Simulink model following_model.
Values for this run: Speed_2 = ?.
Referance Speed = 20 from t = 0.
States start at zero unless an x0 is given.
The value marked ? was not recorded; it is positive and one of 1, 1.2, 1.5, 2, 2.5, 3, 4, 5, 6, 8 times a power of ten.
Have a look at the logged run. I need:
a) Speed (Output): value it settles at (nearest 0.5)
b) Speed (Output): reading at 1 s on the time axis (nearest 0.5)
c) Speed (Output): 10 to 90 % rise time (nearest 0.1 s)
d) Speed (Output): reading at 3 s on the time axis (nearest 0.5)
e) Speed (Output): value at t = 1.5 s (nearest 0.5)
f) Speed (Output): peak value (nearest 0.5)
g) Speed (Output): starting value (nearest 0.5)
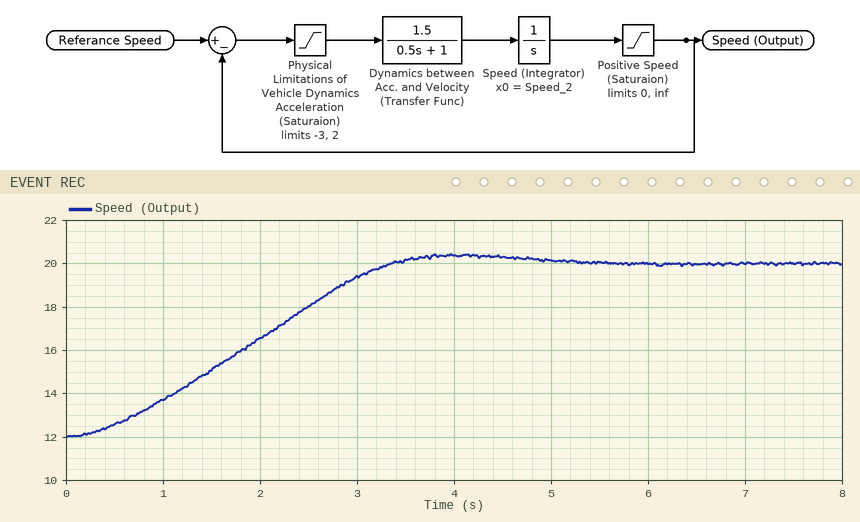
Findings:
20.0
13.5
2.3 s
19.5
15.0
20.5
12.0
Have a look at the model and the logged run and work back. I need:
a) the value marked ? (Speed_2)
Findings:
12
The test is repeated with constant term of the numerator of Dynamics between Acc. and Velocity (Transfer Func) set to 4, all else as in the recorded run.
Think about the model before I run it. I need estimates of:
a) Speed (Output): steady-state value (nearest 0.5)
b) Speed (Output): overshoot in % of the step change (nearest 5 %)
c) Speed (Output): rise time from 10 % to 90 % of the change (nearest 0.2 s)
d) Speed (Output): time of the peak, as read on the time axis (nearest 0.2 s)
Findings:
20.0
15 %
1.0 s
2.0 s
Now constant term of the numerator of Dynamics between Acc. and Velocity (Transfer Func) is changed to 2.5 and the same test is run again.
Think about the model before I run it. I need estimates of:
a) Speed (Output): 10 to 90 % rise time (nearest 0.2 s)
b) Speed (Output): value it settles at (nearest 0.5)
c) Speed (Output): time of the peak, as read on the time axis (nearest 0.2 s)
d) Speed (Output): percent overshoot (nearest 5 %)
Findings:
1.4 s
20.0
2.8 s
10 %
